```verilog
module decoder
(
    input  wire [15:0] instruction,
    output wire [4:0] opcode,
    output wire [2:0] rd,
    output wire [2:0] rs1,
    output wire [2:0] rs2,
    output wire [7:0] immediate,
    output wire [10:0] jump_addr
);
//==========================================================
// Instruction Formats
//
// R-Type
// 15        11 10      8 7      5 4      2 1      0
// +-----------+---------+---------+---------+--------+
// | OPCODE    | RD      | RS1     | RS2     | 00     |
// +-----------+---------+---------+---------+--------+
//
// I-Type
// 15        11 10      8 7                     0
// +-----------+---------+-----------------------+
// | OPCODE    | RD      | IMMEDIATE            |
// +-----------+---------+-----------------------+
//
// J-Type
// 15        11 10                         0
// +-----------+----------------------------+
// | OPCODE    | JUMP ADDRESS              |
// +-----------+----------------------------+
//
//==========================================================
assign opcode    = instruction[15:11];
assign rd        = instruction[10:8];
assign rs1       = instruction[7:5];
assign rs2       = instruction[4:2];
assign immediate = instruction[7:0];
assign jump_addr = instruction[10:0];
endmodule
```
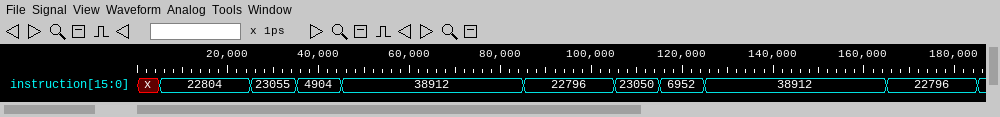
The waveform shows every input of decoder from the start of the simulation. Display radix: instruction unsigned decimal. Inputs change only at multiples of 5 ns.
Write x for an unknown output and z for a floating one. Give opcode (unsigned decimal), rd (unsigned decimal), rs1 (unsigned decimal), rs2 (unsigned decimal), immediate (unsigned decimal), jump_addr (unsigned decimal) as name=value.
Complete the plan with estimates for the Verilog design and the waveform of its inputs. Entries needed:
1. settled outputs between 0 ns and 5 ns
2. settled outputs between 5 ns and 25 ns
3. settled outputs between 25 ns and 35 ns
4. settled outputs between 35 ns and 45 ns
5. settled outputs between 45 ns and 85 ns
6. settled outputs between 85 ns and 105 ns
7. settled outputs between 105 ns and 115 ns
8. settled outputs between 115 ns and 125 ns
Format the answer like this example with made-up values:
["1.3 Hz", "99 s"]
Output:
["opcode=x, rd=x, rs1=x, rs2=x, immediate=x, jump_addr=x", "opcode=11, rd=1, rs1=0, rs2=5, immediate=20, jump_addr=276", "opcode=11, rd=2, rs1=0, rs2=3, immediate=15, jump_addr=527", "opcode=2, rd=3, rs1=1, rs2=2, immediate=40, jump_addr=808", "opcode=19, rd=0, rs1=0, rs2=0, immediate=0, jump_addr=0", "opcode=11, rd=1, rs1=0, rs2=3, immediate=12, jump_addr=268", "opcode=11, rd=2, rs1=0, rs2=2, immediate=10, jump_addr=522", "opcode=3, rd=3, rs1=1, rs2=2, immediate=40, jump_addr=808"]
